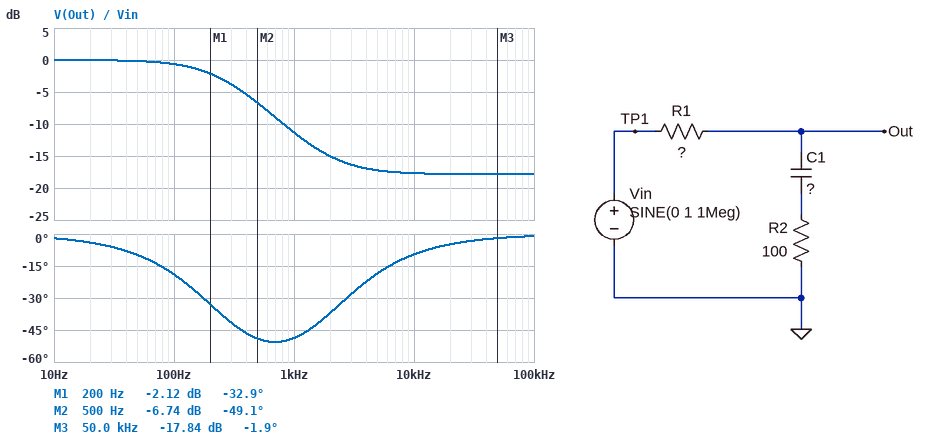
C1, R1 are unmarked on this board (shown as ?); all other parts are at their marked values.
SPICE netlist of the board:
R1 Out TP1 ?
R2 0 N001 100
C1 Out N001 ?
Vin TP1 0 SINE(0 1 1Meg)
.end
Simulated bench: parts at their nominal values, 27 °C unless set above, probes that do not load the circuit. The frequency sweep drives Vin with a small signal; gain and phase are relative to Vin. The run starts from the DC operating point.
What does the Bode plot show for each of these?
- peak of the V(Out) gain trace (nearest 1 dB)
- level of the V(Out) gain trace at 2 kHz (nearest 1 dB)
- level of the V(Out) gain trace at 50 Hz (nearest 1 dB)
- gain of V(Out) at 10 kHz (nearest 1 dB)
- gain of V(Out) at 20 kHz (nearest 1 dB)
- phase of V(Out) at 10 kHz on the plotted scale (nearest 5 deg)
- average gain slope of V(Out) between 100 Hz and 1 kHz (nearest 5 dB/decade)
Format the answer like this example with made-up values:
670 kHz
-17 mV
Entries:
0 dB
-15 dB
0 dB
-18 dB
-18 dB
-10 deg
-10 dB/decade
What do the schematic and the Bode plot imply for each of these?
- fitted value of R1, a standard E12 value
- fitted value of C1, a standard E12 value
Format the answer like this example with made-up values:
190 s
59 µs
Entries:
680 Ω
820 nF
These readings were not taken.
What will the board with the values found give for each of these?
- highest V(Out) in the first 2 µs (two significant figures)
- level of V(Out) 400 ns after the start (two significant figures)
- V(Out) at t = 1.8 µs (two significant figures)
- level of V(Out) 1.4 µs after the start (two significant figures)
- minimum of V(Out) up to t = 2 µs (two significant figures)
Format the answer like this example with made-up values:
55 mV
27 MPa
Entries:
130 mV
76 mV
-120 mV
76 mV
-130 mV
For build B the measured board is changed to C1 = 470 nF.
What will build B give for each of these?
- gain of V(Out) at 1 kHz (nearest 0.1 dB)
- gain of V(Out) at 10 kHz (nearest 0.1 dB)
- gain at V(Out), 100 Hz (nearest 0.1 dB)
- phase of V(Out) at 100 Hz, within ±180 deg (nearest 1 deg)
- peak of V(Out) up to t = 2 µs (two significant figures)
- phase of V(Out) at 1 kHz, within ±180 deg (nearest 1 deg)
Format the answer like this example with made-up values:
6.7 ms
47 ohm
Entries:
-7.6 dB
-17.4 dB
-0.2 dB
-11 deg
130 mV
-50 deg
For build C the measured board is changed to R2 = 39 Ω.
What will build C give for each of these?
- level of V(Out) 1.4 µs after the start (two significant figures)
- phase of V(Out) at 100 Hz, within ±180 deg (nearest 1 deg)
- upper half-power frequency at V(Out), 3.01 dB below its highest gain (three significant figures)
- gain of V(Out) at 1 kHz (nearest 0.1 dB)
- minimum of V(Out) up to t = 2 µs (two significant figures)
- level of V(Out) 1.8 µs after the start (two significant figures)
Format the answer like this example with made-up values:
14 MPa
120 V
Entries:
32 mV
-19 deg
271 Hz
-11.5 dB
-54 mV
-51 mV
